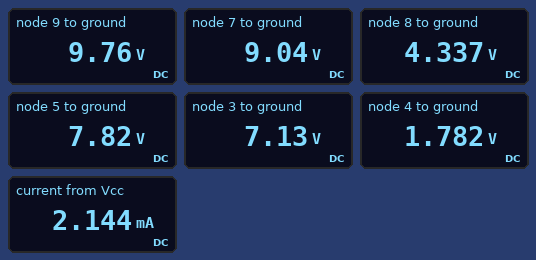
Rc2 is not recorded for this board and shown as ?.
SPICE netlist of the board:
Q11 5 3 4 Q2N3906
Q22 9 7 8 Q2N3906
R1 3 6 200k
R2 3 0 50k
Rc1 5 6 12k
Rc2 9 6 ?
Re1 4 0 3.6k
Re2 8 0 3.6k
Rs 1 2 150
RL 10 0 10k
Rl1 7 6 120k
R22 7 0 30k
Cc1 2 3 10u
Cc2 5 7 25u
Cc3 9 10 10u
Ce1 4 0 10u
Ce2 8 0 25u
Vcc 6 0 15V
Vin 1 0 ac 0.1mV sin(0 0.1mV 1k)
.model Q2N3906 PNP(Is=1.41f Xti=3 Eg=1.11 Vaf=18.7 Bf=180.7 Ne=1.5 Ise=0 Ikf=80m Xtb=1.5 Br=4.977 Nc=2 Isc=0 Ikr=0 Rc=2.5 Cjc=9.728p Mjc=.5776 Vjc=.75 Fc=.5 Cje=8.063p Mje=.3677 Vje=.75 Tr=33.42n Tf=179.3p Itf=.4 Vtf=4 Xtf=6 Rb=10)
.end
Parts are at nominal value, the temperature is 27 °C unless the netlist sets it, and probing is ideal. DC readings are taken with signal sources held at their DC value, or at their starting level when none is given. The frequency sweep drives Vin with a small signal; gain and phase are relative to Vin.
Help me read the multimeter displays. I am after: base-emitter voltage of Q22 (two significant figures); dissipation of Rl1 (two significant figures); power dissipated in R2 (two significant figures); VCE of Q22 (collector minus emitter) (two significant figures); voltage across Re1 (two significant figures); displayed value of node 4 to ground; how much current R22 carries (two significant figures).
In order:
4.7 V
300 µW
1.0 mW
5.4 V
1.8 V
1.782 V
300 µA
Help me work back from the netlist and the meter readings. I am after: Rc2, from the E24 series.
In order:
3.6 kΩ
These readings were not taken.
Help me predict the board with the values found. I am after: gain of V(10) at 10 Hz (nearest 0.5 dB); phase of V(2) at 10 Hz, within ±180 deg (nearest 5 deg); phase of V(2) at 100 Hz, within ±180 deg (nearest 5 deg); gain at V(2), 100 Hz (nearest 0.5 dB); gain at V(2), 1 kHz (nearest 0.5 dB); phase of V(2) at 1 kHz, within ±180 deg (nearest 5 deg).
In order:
-0.5 dB
0 deg
0 deg
0 dB
0 dB
0 deg
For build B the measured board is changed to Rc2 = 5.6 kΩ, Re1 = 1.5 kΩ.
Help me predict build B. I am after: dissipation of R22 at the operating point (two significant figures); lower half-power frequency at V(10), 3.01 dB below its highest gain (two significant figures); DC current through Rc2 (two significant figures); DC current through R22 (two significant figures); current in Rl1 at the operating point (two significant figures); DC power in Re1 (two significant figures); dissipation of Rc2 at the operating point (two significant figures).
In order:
2.0 mW
2.2 Hz
1.2 mA
260 µA
60 µA
370 µW
7.5 mW
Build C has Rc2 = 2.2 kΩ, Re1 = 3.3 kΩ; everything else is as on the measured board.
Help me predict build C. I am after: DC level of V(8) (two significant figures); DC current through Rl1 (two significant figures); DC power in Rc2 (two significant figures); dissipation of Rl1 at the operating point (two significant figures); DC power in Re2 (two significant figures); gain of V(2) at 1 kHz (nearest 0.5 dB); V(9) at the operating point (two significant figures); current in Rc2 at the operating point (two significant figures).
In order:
5.3 V
39 µA
6.9 mW
180 µW
7.8 mW
0 dB
11 V
1.8 mA
